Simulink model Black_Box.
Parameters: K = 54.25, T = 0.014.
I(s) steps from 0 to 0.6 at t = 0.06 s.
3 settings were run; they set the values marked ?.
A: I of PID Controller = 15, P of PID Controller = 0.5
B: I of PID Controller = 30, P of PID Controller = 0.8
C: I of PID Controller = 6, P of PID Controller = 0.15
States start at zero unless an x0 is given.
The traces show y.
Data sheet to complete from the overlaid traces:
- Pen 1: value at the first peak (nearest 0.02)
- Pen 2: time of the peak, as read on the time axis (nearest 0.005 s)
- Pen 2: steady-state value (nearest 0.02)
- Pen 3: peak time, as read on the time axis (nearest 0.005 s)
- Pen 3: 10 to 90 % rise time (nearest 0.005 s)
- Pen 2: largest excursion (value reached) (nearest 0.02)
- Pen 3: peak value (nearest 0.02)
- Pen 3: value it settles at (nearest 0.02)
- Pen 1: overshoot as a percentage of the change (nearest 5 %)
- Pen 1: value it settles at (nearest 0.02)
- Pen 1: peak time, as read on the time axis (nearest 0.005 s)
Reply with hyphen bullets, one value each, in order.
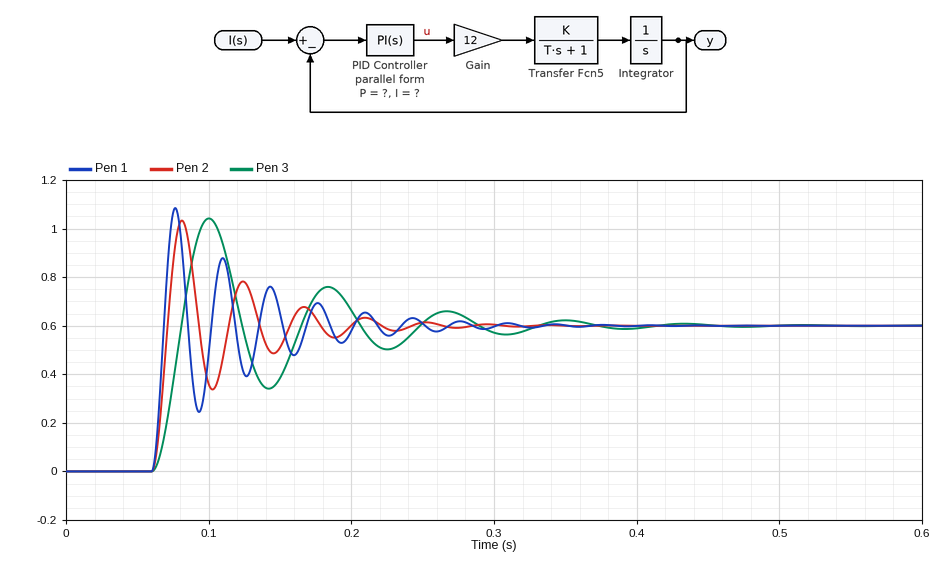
- 1.08
- 0.080 s
- 0.60
- 0.100 s
- 0.015 s
- 1.04
- 1.04
- 0.60
- 80 %
- 0.60
- 0.075 s
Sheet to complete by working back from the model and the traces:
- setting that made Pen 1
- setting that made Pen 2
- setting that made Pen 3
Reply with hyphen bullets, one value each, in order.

- B
- A
- C
